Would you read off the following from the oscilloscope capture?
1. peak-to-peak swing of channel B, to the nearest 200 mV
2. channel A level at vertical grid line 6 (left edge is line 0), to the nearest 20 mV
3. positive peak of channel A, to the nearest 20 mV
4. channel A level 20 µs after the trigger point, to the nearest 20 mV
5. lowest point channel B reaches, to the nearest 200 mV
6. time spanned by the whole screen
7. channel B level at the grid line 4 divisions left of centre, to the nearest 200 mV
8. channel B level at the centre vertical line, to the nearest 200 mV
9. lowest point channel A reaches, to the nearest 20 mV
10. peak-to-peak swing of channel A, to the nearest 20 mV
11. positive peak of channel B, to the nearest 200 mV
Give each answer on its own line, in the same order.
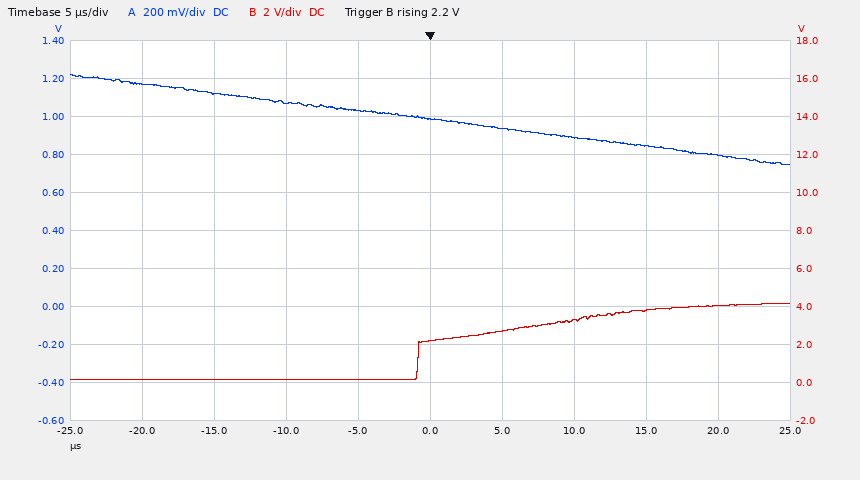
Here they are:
4.0 V
940 mV
1.22 V
800 mV
200 mV
50 µs
200 mV
2.2 V
740 mV
480 mV
4.2 V
